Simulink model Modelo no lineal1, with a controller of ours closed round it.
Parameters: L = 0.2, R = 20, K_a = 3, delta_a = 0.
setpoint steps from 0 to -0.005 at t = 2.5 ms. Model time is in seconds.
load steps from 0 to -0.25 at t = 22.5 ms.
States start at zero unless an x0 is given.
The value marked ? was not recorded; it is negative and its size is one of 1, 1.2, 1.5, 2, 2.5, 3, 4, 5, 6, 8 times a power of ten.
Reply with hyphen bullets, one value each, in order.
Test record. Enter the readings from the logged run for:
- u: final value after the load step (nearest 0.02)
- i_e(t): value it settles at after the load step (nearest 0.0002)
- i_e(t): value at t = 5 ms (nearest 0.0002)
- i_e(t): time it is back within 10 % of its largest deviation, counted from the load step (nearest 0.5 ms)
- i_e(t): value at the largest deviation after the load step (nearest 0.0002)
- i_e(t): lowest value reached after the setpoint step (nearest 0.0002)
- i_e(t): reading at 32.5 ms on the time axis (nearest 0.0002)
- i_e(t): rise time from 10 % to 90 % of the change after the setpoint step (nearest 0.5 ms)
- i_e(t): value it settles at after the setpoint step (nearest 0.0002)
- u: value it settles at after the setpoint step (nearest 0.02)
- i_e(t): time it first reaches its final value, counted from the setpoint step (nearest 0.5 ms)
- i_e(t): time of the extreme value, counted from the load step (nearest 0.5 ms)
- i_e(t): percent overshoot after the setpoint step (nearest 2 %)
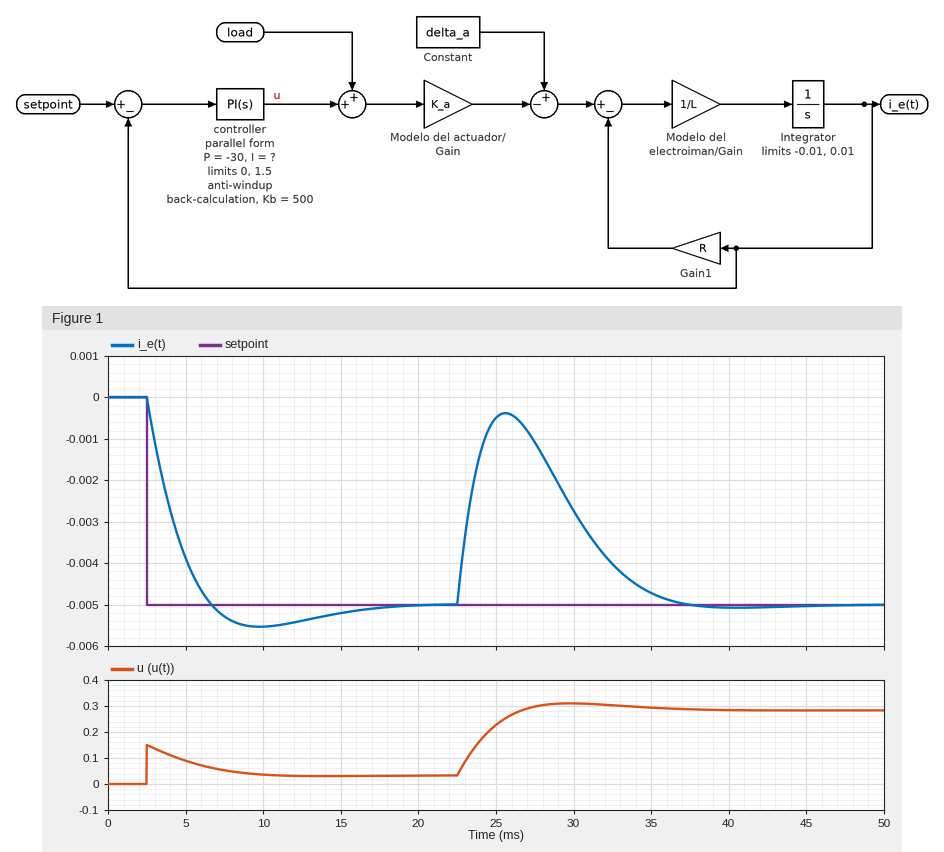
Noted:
- 0.28
- -0.0050
- -0.0038
- 11.5 ms
- -0.0004
- -0.0056
- -0.0040
- 3.0 ms
- -0.0050
- 0.04
- 4.0 ms
- 3.0 ms
- 10 %
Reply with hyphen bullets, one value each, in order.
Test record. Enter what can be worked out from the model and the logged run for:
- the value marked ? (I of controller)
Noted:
- -8000
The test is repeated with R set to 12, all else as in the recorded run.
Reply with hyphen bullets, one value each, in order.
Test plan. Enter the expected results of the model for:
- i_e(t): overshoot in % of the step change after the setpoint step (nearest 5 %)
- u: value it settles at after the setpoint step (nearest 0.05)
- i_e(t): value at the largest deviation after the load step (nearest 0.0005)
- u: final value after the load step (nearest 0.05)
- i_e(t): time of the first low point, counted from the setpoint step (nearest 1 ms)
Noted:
- 15 %
- 0.00
- 0.0000
- 0.25
- 7 ms
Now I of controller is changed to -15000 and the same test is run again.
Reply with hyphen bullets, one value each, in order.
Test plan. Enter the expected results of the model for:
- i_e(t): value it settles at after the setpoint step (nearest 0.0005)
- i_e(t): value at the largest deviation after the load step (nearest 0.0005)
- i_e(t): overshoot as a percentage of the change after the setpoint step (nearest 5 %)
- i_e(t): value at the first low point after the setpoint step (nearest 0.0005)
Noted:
- -0.0050
- -0.0010
- 20 %
- -0.0060
